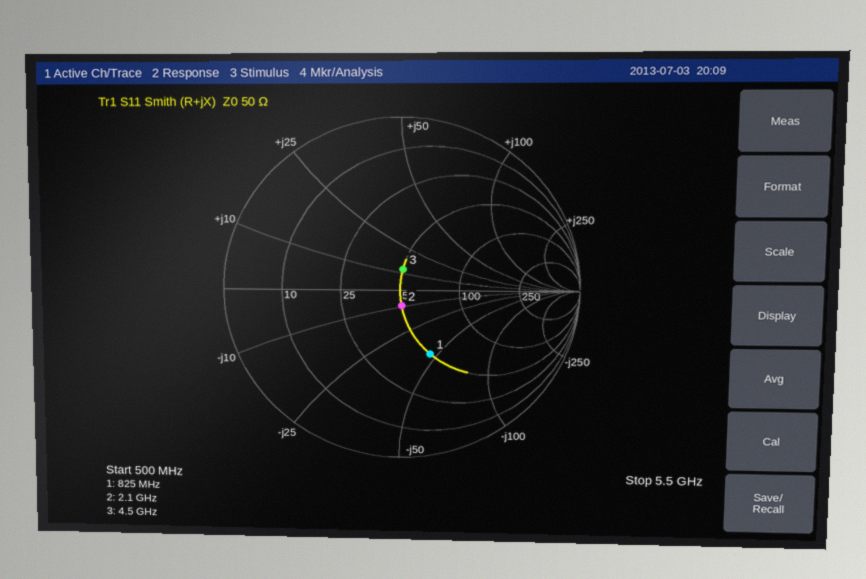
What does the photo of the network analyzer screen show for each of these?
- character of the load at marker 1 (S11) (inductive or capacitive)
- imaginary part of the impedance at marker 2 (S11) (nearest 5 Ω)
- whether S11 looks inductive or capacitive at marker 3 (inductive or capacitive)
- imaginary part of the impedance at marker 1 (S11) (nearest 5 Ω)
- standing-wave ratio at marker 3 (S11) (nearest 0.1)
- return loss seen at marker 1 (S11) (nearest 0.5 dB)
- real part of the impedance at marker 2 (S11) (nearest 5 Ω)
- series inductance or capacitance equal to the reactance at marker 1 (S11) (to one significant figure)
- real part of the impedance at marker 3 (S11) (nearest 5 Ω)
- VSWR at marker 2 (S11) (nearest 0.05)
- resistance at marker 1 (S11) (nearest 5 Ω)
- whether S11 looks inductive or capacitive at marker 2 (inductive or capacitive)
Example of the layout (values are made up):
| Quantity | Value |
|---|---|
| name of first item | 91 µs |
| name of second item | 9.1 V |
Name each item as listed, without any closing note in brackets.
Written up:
| Quantity | Value |
|---|---|
| character of the load at marker 1 (S11) | capacitive |
| imaginary part of the impedance at marker 2 (S11) | -10 Ω |
| whether S11 looks inductive or capacitive at marker 3 | inductive |
| imaginary part of the impedance at marker 1 (S11) | -45 Ω |
| standing-wave ratio at marker 3 (S11) | 1.3 |
| return loss seen at marker 1 (S11) | 7.5 dB |
| real part of the impedance at marker 2 (S11) | 50 Ω |
| series inductance or capacitance equal to the reactance at marker 1 (S11) | 4 pF |
| real part of the impedance at marker 3 (S11) | 50 Ω |
| VSWR at marker 2 (S11) | 1.20 |
| resistance at marker 1 (S11) | 50 Ω |
| whether S11 looks inductive or capacitive at marker 2 | capacitive |
